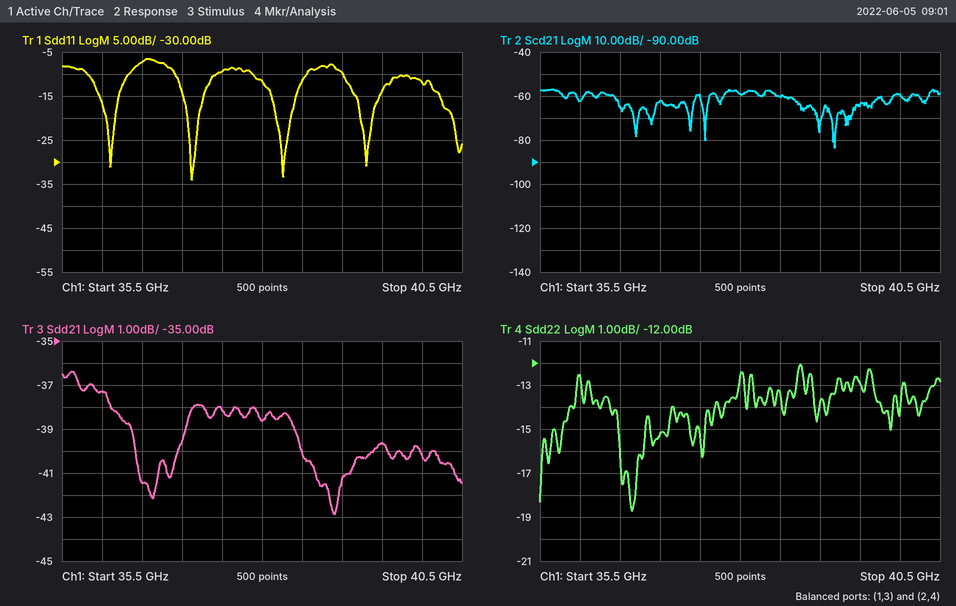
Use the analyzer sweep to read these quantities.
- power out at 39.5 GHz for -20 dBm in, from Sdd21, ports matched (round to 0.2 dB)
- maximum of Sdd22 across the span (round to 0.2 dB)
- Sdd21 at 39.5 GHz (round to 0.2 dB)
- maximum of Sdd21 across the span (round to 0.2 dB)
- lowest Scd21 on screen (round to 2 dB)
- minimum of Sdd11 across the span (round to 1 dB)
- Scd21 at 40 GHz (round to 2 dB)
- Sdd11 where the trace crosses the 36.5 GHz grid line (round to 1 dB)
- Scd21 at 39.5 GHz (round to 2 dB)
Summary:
-59.6 dBm
-12.0 dB
-39.6 dB
-36.4 dB
-84 dB
-34 dB
-60 dB
-7 dB
-64 dB
